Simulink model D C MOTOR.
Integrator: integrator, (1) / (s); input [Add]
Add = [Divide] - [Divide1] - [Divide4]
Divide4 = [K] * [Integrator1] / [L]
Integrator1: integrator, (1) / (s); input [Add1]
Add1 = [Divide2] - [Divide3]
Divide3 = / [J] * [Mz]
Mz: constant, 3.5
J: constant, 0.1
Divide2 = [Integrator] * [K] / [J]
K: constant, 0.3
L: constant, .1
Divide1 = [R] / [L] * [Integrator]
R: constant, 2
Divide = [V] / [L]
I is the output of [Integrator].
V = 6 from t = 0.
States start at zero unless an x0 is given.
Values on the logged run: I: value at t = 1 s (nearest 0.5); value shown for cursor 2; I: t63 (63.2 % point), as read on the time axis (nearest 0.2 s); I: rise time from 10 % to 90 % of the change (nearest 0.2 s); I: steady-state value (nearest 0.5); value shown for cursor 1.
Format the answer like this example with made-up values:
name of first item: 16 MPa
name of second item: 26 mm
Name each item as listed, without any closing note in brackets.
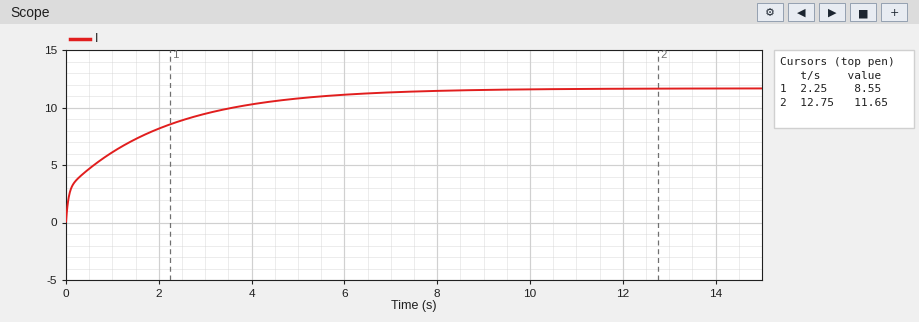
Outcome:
I: value at t = 1 s: 6.0
value shown for cursor 2: 11.65
I: t63 (63.2 % point), as read on the time axis: 1.6 s
I: rise time from 10 % to 90 % of the change: 4.4 s
I: steady-state value: 11.5
value shown for cursor 1: 8.55
